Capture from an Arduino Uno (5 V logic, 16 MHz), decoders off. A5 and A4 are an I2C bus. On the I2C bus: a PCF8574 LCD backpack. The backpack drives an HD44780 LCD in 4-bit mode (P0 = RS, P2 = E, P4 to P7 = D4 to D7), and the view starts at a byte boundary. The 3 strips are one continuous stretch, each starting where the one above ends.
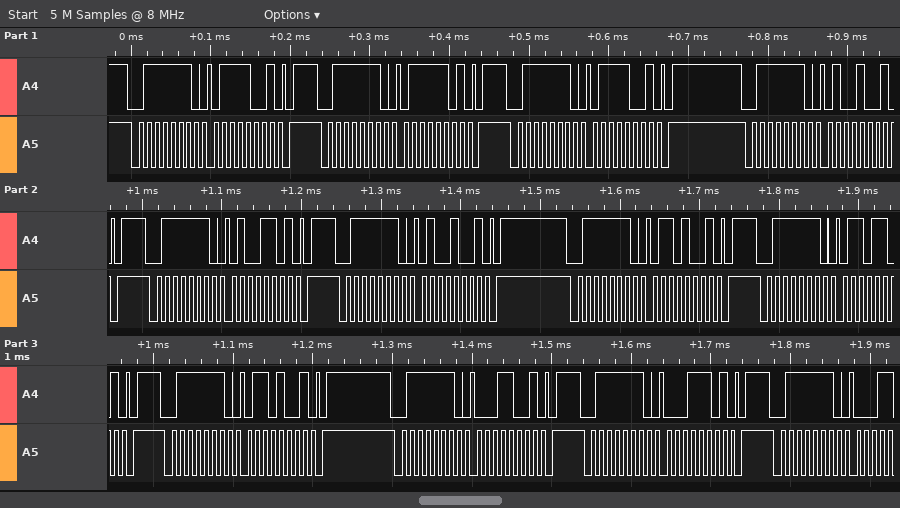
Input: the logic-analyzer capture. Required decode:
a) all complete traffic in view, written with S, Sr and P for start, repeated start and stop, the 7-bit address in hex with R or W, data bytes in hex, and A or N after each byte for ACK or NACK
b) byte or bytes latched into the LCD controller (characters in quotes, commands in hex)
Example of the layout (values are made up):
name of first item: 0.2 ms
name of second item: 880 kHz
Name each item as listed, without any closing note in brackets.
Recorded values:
all complete traffic in view, written with S, Sr and P for start, repeated start and stop, the 7-bit address in hex with R or W, data bytes in hex, and A or N after each byte for ACK or NACK: S 3FW A 79 A P S 3FW A 7D A P S 3FW A 79 A P S 3FW A 49 A P S 3FW A 4D A P S 3FW A 49 A P S 3FW A 69 A P S 3FW A 6D A P S 3FW A 69 A P S 3FW A 19 A P S 3FW A 1D A P S 3FW A
byte or bytes latched into the LCD controller: 't'
